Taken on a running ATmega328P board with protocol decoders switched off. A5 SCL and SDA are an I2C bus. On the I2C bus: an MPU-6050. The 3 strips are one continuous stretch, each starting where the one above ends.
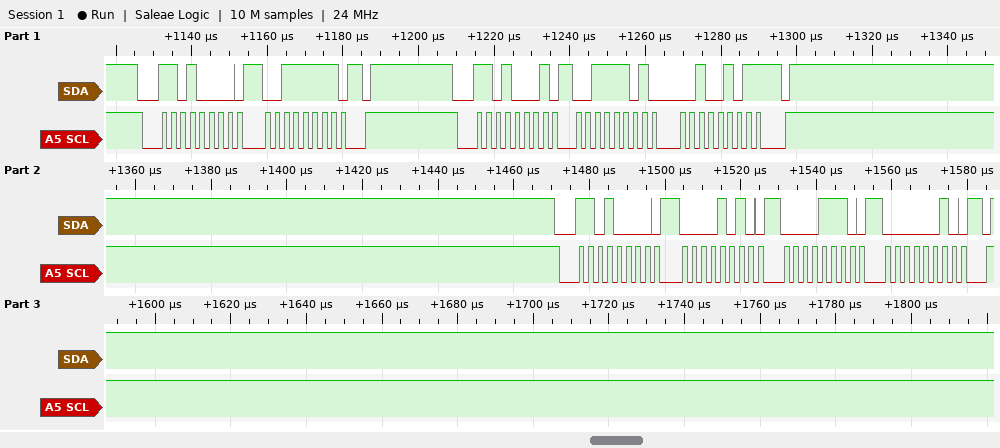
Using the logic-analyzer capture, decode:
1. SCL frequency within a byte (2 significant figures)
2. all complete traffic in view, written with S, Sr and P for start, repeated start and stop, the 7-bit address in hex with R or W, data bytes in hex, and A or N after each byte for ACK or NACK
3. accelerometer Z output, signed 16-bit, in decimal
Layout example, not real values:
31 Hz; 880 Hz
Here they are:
400 kHz; S 68W A 3F A P S 68R A 3D A 25 N P S 68W A 0A A 0E A 02 A P; 15653
